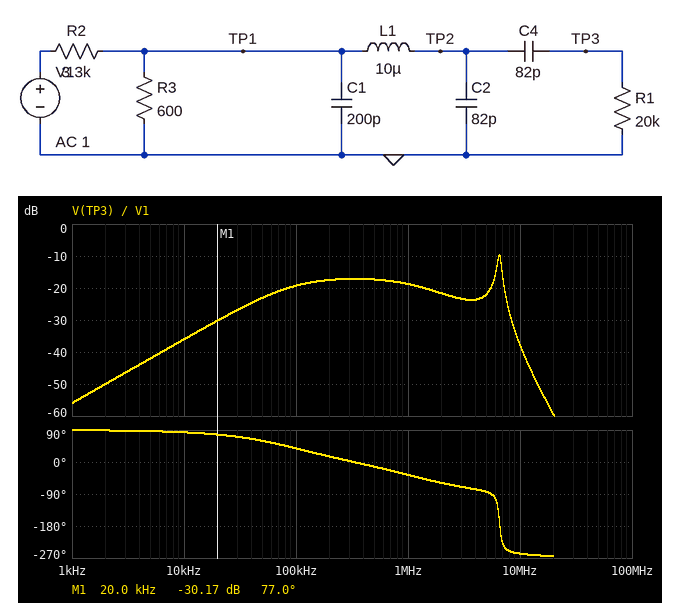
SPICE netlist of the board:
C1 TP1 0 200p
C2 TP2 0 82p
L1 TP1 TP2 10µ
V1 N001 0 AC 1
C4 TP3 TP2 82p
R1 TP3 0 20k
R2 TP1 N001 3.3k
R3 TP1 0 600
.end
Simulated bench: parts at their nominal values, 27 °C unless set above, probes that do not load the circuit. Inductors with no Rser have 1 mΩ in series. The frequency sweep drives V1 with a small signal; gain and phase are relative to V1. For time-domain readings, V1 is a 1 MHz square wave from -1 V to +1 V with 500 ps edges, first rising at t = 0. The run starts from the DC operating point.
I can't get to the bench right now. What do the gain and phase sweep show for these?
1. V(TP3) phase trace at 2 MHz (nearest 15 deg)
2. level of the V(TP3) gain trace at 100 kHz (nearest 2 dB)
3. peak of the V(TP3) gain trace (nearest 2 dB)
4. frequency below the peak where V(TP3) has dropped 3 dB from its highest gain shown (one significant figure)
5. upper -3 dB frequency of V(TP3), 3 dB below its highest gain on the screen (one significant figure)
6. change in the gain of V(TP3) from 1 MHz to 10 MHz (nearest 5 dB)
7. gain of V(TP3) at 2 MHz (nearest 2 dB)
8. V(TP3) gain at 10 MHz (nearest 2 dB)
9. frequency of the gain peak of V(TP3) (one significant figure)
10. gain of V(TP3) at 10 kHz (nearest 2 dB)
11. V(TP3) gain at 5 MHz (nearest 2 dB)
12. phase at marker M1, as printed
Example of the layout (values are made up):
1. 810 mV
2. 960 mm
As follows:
1. -60 deg
2. -20 dB
3. -10 dB
4. 6 MHz
5. 7 MHz
6. -20 dB
7. -22 dB
8. -38 dB
9. 7 MHz
10. -36 dB
11. -22 dB
12. 77.0 deg
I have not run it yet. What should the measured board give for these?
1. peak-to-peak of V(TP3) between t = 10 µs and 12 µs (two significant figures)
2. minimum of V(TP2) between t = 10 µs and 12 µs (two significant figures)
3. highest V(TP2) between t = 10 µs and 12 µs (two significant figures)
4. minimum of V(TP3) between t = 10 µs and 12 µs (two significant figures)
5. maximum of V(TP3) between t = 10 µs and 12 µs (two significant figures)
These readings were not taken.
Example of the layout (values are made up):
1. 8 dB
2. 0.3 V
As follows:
1. 310 mV
2. -160 mV
3. 160 mV
4. -160 mV
5. 160 mV
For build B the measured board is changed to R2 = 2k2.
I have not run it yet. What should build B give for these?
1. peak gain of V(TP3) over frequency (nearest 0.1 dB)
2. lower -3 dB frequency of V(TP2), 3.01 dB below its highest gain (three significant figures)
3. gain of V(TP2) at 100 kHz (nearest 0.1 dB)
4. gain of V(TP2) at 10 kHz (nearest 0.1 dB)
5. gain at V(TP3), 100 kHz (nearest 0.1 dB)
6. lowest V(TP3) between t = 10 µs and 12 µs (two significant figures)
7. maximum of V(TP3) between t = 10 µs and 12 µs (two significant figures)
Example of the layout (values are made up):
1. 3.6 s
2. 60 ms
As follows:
1. -6.6 dB
2. 6.24 MHz
3. -13.5 dB
4. -13.4 dB
5. -16.4 dB
6. -220 mV
7. 220 mV
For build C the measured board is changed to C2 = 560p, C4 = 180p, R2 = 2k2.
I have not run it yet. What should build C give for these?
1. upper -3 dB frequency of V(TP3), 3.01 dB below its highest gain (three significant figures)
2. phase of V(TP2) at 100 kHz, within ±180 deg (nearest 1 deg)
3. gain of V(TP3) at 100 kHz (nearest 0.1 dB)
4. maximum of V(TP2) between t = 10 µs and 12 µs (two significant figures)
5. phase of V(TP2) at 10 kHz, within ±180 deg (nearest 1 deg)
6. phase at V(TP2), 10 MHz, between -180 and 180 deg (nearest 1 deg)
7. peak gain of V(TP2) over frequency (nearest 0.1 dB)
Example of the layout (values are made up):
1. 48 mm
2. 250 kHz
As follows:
1. 568 kHz
2. -13 deg
3. -14.5 dB
4. 130 mV
5. -2 deg
6. 101 deg
7. -13.4 dB
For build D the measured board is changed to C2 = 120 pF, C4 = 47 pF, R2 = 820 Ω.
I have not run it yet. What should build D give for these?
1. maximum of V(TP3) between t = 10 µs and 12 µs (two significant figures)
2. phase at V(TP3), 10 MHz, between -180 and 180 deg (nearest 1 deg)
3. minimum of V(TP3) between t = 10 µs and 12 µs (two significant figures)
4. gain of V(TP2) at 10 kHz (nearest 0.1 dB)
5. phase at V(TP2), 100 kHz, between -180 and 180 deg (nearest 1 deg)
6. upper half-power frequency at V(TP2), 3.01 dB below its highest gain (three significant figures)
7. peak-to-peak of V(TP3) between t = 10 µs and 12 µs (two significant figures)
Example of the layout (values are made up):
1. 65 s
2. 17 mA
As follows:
1. 460 mV
2. 107 deg
3. -460 mV
4. -7.5 dB
5. -4 deg
6. 6.04 MHz
7. 920 mV
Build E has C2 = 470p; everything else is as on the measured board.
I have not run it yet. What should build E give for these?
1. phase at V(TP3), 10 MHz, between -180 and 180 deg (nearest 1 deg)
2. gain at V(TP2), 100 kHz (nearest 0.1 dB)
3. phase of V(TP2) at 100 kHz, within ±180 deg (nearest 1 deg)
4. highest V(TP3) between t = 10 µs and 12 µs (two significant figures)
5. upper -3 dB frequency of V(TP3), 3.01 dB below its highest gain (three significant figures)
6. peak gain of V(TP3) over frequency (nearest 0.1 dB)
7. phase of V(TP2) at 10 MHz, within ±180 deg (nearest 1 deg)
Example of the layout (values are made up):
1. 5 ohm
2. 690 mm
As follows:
1. 101 deg
2. -16.6 dB
3. -13 deg
4. 93 mV
5. 687 kHz
6. -18.0 dB
7. 100 deg
